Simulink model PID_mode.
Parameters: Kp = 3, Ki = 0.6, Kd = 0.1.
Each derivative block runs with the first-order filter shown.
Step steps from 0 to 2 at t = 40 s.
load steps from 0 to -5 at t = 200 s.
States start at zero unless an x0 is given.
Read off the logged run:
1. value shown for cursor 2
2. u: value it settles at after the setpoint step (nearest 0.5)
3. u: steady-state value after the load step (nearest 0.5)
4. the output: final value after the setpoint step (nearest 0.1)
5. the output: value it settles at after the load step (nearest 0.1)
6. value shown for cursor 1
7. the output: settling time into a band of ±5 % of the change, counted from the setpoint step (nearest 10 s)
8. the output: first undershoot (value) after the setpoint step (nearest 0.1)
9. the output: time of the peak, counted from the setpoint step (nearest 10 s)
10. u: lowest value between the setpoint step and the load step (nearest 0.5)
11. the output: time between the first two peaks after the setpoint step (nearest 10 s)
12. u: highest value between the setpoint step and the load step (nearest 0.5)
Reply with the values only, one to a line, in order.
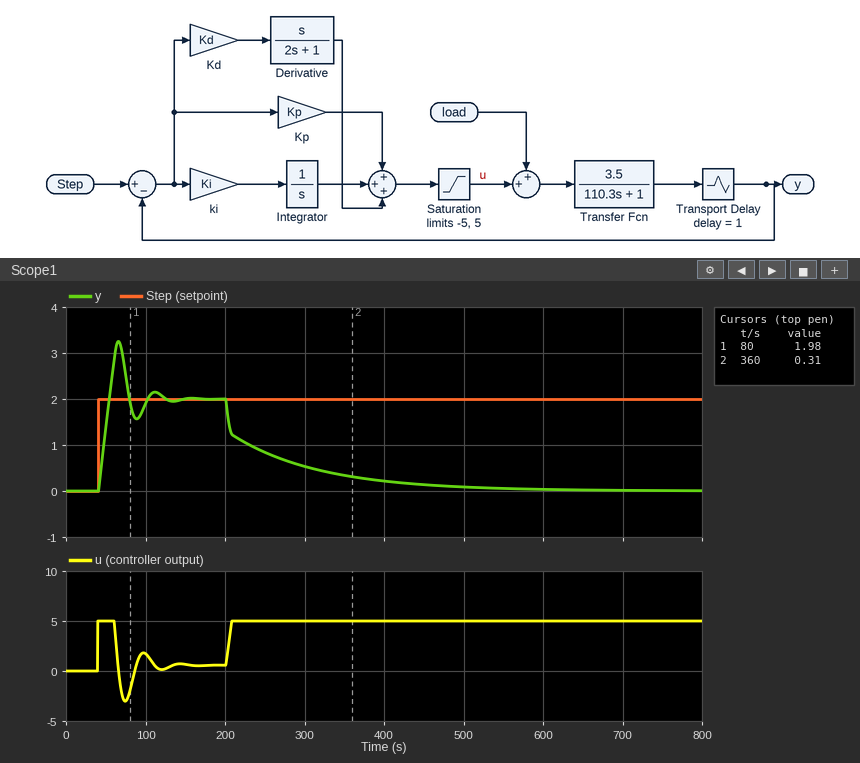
0.31
0.5
5.0
2.0
0.0
1.98
80 s
1.6
30 s
-3.0
50 s
5.0
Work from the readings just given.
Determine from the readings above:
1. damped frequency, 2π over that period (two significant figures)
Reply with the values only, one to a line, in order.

0.13 rad/s
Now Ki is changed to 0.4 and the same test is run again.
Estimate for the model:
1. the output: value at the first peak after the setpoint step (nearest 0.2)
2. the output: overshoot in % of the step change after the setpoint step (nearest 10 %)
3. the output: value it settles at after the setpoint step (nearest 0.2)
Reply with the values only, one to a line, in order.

3.0
50 %
2.0
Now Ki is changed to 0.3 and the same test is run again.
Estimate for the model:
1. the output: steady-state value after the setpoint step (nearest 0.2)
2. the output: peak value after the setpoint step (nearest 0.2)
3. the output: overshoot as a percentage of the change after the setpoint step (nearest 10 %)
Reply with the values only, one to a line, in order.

2.0
2.8
40 %
